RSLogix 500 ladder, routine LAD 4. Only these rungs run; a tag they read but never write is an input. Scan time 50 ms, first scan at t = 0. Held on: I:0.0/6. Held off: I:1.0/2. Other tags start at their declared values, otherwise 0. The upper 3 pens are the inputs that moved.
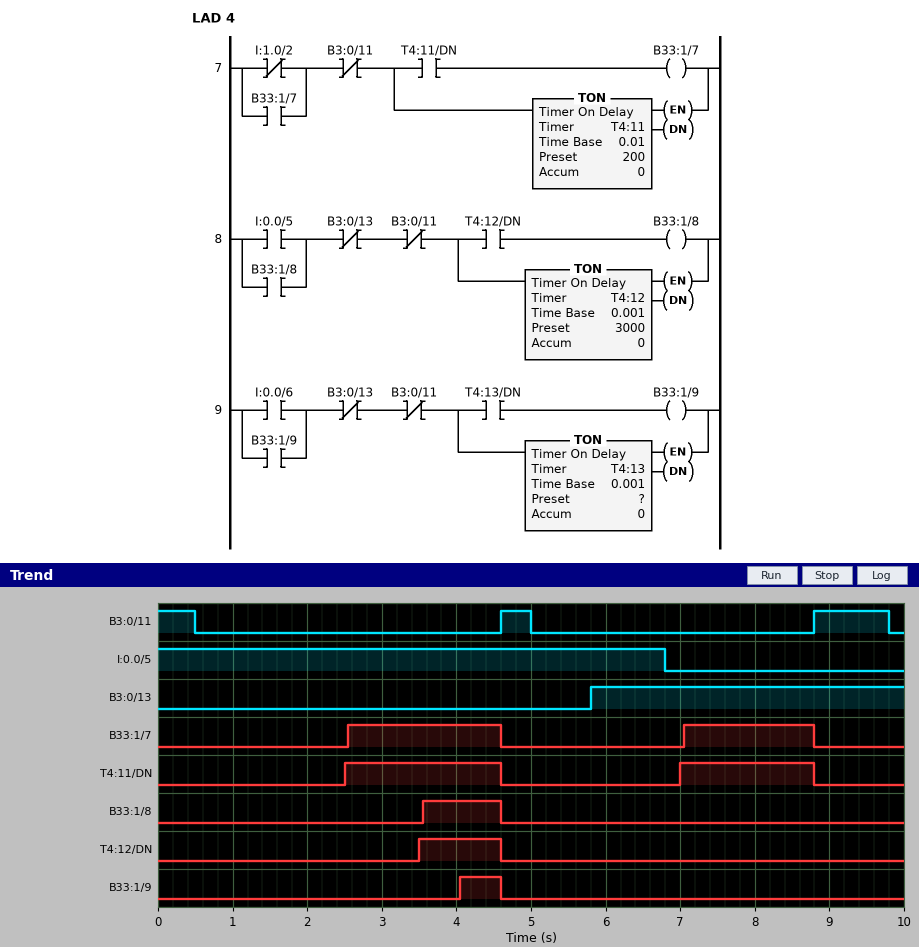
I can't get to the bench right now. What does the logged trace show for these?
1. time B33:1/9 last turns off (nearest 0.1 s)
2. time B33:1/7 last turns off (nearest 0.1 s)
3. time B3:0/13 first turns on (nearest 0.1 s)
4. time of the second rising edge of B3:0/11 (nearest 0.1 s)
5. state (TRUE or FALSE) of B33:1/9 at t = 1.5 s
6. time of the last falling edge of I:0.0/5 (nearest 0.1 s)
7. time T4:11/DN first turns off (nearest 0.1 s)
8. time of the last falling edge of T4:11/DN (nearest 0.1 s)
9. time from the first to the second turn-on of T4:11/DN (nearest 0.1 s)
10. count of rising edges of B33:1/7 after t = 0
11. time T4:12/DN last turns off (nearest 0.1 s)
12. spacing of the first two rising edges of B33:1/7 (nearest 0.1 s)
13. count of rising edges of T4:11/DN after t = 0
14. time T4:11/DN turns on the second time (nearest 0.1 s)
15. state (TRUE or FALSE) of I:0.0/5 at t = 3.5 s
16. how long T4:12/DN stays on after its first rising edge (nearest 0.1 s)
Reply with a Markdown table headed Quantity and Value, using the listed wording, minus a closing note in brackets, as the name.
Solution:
| Quantity | Value |
|---|---|
| time B33:1/9 last turns off | 4.6 s |
| time B33:1/7 last turns off | 8.8 s |
| time B3:0/13 first turns on | 5.8 s |
| time of the second rising edge of B3:0/11 | 8.8 s |
| state (TRUE or FALSE) of B33:1/9 at t = 1.5 s | FALSE |
| time of the last falling edge of I:0.0/5 | 6.8 s |
| time T4:11/DN first turns off | 4.6 s |
| time of the last falling edge of T4:11/DN | 8.8 s |
| time from the first to the second turn-on of T4:11/DN | 4.5 s |
| count of rising edges of B33:1/7 after t = 0 | 2 |
| time T4:12/DN last turns off | 4.6 s |
| spacing of the first two rising edges of B33:1/7 | 4.5 s |
| count of rising edges of T4:11/DN after t = 0 | 2 |
| time T4:11/DN turns on the second time | 7.0 s |
| state (TRUE or FALSE) of I:0.0/5 at t = 3.5 s | TRUE |
| how long T4:12/DN stays on after its first rising edge | 1.1 s |
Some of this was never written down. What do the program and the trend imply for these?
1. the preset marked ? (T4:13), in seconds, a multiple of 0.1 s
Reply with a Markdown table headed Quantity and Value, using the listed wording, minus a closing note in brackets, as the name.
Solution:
| Quantity | Value |
|---|---|
| the preset marked ? (T4:13), in seconds, a multiple of 0.1 s | 3.5 s |
